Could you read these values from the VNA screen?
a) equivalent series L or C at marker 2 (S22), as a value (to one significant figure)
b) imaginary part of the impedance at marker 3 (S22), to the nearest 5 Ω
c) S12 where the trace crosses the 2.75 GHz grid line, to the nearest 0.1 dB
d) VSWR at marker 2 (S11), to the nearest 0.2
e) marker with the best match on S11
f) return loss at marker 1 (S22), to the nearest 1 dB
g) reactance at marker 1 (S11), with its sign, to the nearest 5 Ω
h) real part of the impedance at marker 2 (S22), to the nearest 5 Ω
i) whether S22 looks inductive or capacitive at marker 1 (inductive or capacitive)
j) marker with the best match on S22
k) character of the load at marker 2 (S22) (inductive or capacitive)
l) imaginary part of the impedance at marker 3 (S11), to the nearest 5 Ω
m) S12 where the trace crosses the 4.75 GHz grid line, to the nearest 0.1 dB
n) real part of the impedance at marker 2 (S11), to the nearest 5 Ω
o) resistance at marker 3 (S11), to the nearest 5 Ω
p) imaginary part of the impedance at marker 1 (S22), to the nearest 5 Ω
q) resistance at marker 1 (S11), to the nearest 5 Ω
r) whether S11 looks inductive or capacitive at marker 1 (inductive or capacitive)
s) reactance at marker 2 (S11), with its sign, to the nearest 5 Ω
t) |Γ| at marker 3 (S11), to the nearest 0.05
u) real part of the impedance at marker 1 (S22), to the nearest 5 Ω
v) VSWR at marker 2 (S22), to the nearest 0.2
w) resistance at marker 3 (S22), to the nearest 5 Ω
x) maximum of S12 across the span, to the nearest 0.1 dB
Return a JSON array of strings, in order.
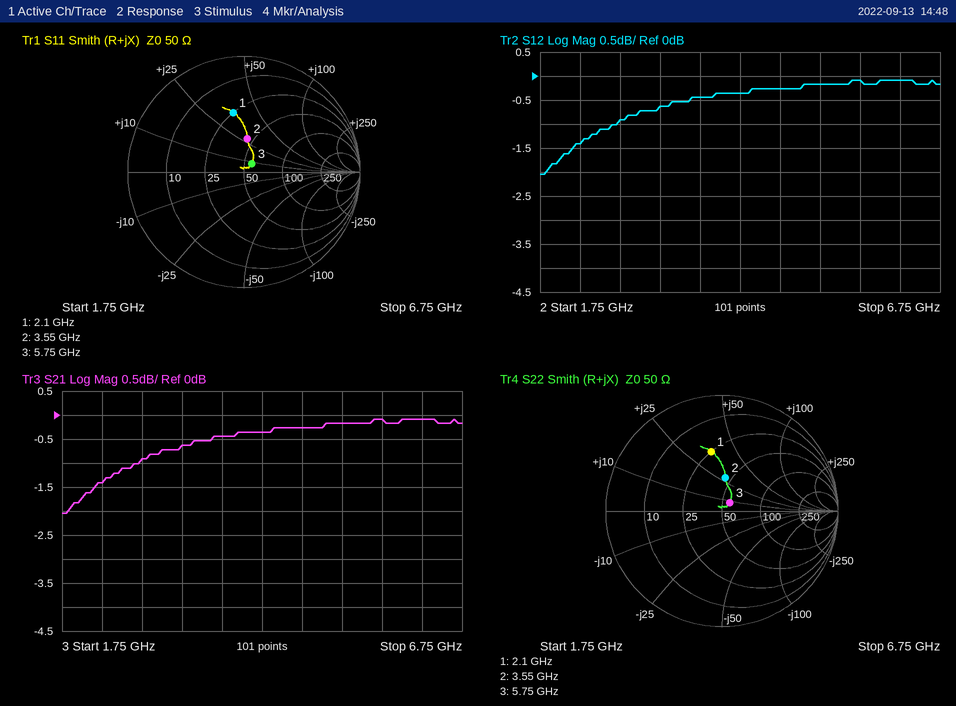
["1 nH", "+10 Ω", "-0.9 dB", "1.8", "marker 3", "6 dB", "+35 Ω", "45 Ω", "inductive", "marker 3", "inductive", "+10 Ω", "-0.3 dB", "45 Ω", "55 Ω", "+35 Ω", "25 Ω", "inductive", "+30 Ω", "0.10", "25 Ω", "1.8", "55 Ω", "-0.1 dB"]
